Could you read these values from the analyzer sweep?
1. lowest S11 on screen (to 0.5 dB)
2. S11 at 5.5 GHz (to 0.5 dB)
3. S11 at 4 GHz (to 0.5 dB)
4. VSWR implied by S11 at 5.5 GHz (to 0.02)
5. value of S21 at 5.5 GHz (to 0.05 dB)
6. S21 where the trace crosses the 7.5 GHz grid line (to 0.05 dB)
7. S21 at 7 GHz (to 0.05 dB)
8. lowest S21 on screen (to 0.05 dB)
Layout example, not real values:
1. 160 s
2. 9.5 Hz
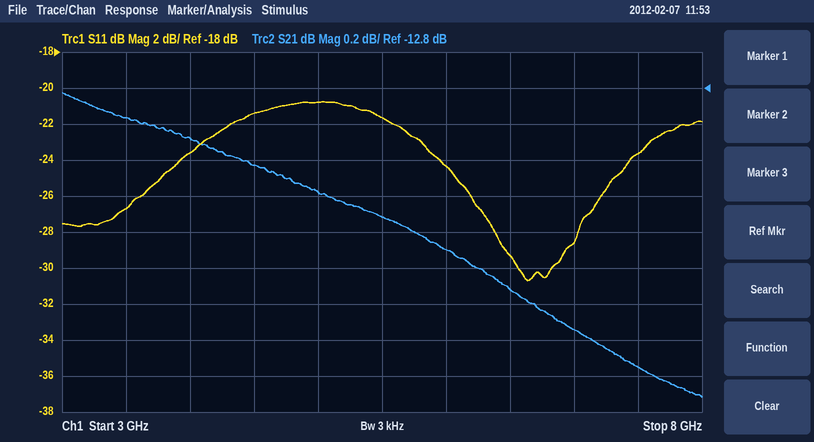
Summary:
1. -30.5 dB
2. -21.5 dB
3. -23.5 dB
4. 1.18
5. -13.50 dB
6. -14.35 dB
7. -14.15 dB
8. -14.50 dB
